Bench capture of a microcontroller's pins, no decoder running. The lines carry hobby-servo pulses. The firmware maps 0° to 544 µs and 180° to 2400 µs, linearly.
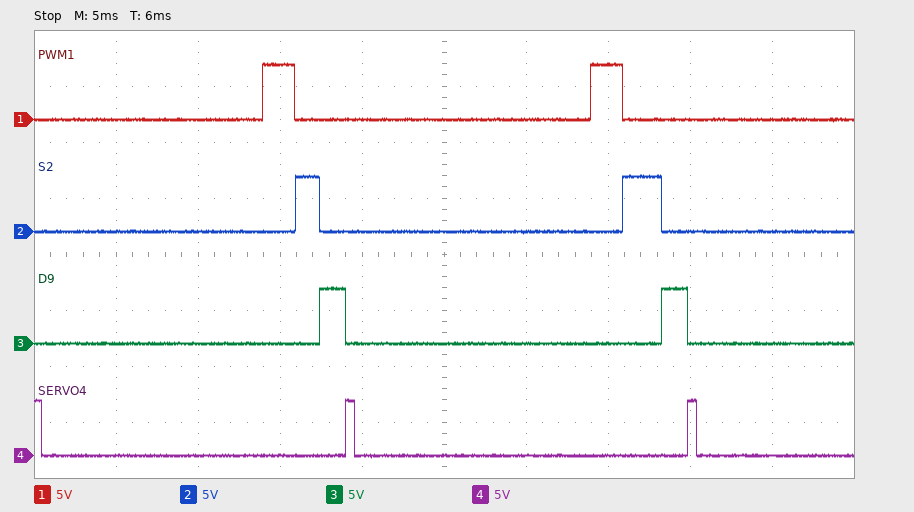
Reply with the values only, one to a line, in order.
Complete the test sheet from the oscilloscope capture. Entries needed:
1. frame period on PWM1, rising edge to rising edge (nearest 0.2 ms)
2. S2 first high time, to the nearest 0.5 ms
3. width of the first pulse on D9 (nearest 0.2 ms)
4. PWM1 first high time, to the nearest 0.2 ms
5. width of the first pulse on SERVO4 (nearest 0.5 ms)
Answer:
20.0 ms
1.5 ms
1.6 ms
2.0 ms
0.5 ms
